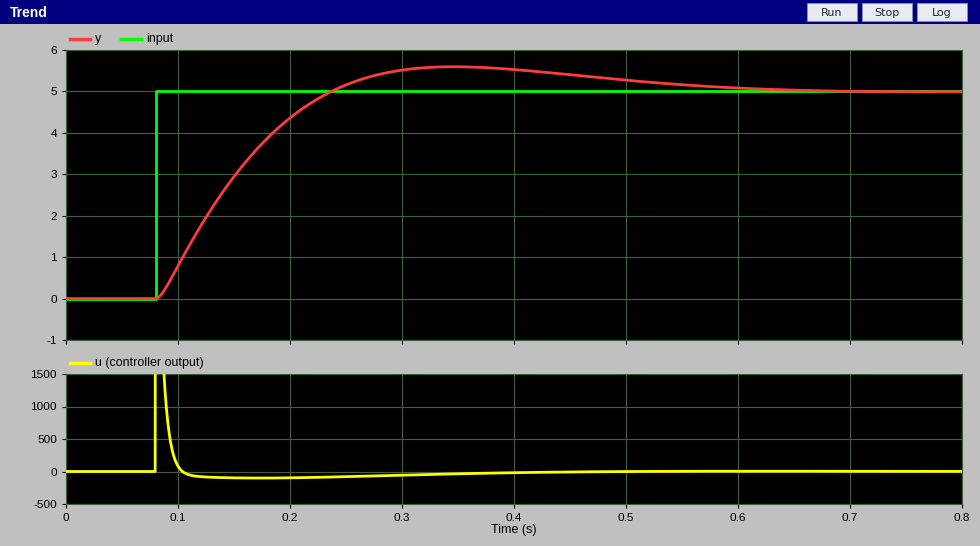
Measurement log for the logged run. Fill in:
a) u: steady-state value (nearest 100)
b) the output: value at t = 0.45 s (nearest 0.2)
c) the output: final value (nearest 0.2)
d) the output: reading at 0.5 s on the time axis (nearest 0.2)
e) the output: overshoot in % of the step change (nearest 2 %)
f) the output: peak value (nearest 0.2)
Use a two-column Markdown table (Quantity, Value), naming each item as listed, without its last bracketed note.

| Quantity | Value |
|---|---|
| u: steady-state value | 0 |
| the output: value at t = 0.45 s | 5.4 |
| the output: final value | 5.0 |
| the output: reading at 0.5 s on the time axis | 5.2 |
| the output: overshoot in % of the step change | 12 % |
| the output: peak value | 5.6 |
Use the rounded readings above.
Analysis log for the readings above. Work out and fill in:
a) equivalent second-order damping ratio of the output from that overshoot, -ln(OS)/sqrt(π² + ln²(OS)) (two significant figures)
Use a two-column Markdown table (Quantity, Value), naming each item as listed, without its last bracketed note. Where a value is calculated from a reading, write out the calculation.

| Quantity | Value |
|---|---|
| equivalent second-order damping ratio of the output from that overshoot, -ln(OS)/sqrt(π² + ln²(OS)) | ln(0.12) = -2.120; 2.120 / sqrt(9.870 + 4.496) = 0.56 |
